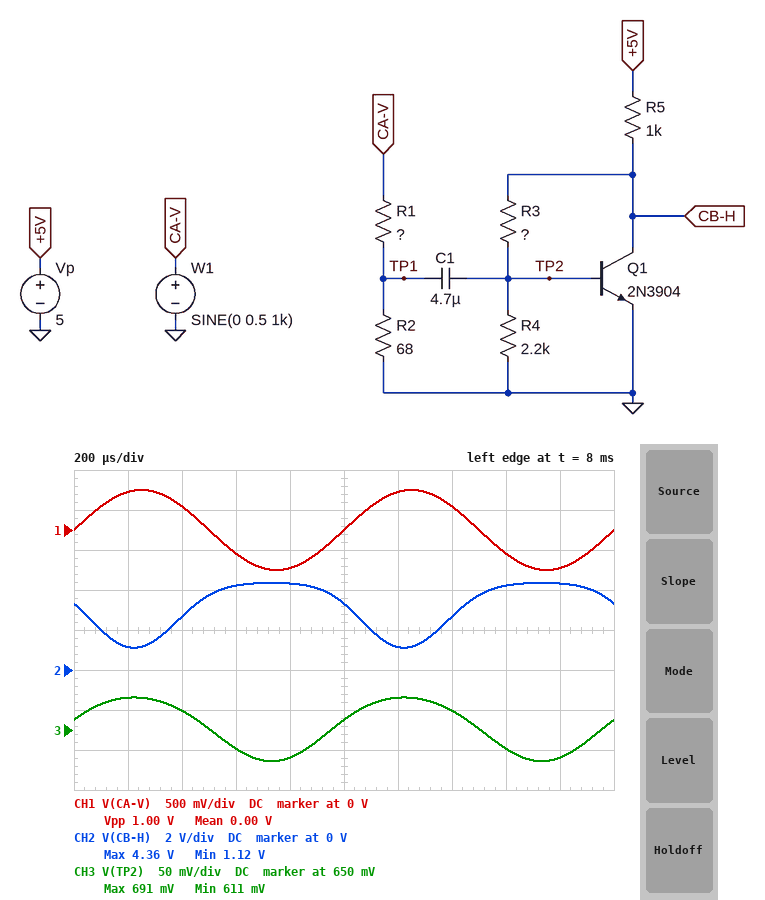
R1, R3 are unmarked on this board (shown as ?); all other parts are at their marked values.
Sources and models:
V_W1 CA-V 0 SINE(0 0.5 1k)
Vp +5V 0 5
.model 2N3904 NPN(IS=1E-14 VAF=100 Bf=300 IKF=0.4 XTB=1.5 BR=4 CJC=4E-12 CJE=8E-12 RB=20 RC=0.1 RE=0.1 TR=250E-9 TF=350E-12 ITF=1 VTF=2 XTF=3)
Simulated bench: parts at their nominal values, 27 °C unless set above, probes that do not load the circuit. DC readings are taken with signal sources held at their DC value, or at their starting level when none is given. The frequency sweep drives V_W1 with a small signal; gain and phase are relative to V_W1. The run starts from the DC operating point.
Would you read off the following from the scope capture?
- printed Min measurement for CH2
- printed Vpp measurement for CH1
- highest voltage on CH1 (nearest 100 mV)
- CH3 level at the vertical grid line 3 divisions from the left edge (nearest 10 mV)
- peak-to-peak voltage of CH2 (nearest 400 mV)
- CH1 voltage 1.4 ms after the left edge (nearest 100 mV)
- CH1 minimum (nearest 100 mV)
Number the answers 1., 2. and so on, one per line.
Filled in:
1. 1.12 V
2. 1.00 V
3. 500 mV
4. 630 mV
5. 3.2 V
6. 300 mV
7. -500 mV
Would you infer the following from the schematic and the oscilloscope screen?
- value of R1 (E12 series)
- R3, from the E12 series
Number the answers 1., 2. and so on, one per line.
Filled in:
1. 560 Ω
2. 8.2 kΩ
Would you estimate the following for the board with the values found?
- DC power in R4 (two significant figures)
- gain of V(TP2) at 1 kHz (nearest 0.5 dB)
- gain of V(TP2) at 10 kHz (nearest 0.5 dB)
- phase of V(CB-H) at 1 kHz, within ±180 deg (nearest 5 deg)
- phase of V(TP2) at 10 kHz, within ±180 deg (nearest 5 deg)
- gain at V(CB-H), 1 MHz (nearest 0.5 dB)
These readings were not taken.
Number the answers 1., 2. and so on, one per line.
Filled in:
1. 200 µW
2. -22.5 dB
3. -22.5 dB
4. -170 deg
5. 0 deg
6. 11.5 dB
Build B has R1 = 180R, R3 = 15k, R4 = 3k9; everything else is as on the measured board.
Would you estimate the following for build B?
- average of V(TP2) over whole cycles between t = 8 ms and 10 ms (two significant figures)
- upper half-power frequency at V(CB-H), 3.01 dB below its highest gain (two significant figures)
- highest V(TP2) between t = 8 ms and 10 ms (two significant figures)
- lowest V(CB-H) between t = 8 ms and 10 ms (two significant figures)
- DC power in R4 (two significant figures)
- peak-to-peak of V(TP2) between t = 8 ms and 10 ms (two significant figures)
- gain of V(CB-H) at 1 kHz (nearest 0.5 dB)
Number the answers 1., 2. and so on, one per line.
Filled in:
1. 590 mV
2. 14 MHz
3. 710 mV
4. 51 mV
5. 110 µW
6. 240 mV
7. 21.5 dB
